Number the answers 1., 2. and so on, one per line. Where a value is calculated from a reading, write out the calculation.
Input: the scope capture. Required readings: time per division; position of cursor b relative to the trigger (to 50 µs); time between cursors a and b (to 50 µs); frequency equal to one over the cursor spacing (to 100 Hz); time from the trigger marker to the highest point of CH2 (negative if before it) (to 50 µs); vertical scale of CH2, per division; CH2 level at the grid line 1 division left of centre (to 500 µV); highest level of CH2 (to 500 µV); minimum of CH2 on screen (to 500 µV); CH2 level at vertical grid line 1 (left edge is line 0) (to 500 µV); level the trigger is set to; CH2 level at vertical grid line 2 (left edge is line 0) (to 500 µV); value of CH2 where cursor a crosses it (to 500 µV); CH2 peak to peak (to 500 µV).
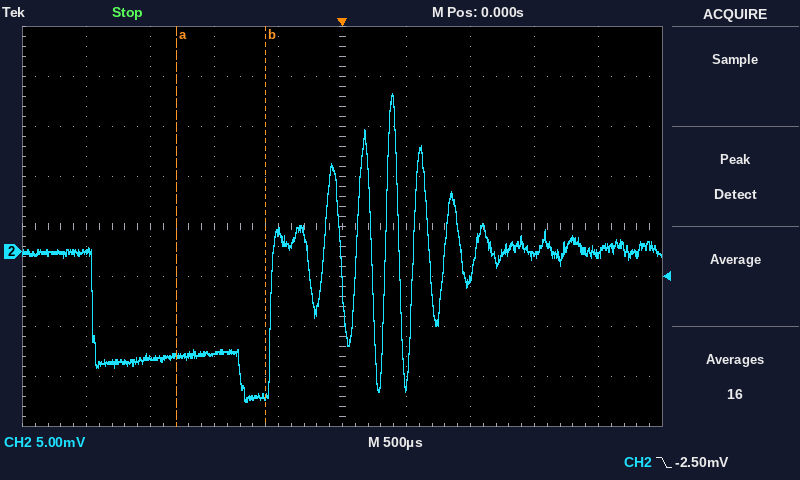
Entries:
1. 500 µs
2. -600 µs
3. 700 µs
4. 1 / 700 µs ≈ 1.4 kHz
5. +400 µs
6. 5 mV
7. 2.0 mV
8. 16.0 mV
9. -15.0 mV
10. 0.0 mV
11. -2.50 mV
12. -10.5 mV
13. -10.5 mV
14. 16.0 mV − (-15.0 mV) = 31.0 mV
